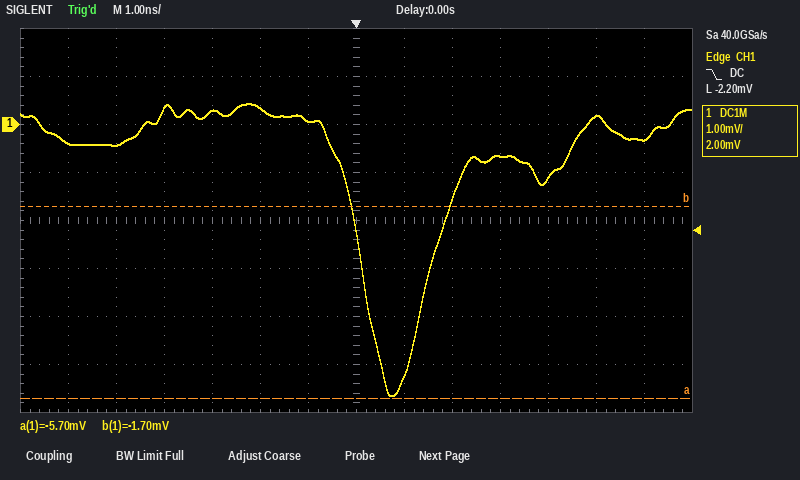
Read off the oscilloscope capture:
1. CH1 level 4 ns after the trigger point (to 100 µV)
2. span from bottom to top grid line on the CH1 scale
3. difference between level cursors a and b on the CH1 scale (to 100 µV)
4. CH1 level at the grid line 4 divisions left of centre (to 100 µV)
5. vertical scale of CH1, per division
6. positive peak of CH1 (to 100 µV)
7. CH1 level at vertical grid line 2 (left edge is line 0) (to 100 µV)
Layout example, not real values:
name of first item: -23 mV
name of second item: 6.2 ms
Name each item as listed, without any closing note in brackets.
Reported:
CH1 level 4 ns after the trigger point: -1.1 mV
span from bottom to top grid line on the CH1 scale: 8 mV
difference between level cursors a and b on the CH1 scale: 4.0 mV
CH1 level at the grid line 4 divisions left of centre: 300 µV
vertical scale of CH1, per division: 1 mV
positive peak of CH1: 400 µV
CH1 level at vertical grid line 2 (left edge is line 0): -400 µV
